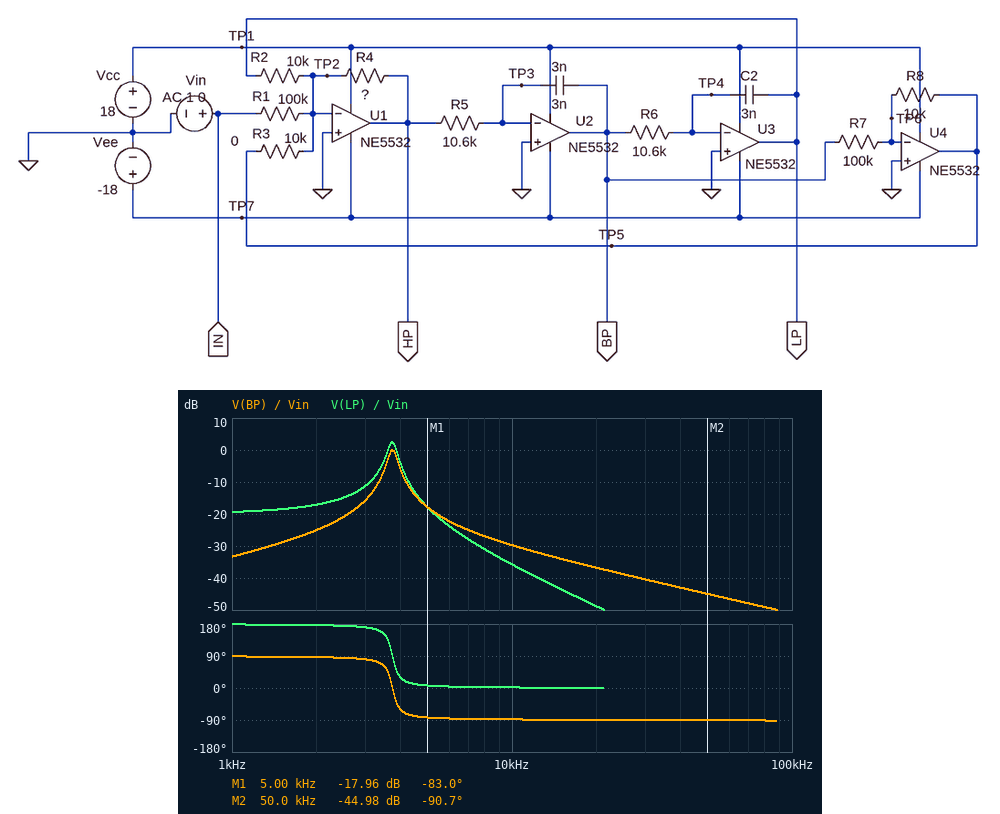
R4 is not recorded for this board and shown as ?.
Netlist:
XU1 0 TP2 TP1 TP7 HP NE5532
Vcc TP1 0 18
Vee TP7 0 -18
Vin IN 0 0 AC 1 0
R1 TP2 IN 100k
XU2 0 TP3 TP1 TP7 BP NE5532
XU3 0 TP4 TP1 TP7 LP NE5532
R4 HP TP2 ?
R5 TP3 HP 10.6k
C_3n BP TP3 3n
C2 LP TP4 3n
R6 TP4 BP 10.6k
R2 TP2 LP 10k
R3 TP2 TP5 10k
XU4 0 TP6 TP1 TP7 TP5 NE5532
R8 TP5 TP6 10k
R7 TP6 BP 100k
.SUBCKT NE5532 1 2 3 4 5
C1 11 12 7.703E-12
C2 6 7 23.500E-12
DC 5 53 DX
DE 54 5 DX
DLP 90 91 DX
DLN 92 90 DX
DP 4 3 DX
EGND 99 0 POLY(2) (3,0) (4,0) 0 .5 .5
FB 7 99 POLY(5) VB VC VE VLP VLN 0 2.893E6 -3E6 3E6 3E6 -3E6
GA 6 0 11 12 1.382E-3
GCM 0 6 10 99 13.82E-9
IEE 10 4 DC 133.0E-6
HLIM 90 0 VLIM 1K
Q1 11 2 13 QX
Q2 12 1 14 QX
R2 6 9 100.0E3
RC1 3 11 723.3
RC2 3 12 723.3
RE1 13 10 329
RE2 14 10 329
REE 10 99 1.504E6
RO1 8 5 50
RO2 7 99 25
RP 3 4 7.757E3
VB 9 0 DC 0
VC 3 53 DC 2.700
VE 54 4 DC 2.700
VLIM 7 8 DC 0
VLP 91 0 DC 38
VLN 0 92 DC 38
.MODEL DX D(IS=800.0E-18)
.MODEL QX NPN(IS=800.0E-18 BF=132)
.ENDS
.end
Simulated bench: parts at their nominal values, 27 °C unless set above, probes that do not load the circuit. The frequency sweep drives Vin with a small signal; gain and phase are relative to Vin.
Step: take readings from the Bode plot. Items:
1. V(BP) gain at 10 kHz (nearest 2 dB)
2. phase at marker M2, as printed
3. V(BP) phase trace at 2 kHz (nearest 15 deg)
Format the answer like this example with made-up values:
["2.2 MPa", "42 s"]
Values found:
["-30 dB", "-90.7 deg", "90 deg"]
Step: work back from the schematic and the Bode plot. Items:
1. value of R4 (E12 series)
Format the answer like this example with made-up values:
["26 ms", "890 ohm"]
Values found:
["5.6 kΩ"]
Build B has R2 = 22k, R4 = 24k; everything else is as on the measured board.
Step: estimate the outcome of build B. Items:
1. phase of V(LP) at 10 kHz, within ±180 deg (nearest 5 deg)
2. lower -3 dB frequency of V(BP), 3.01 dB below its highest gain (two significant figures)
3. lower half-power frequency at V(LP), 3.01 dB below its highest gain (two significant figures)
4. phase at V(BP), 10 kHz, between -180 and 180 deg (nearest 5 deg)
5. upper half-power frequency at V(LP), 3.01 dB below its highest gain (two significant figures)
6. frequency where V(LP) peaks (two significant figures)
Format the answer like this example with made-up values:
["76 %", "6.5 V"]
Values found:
["10 deg", "4.7 kHz", "4.5 kHz", "-80 deg", "5.7 kHz", "5.2 kHz"]
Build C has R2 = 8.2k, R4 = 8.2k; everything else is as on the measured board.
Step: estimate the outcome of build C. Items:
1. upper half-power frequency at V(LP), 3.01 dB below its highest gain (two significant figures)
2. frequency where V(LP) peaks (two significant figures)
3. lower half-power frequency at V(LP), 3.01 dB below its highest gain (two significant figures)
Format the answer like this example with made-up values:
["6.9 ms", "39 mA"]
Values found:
["5.2 kHz", "5.0 kHz", "4.8 kHz"]
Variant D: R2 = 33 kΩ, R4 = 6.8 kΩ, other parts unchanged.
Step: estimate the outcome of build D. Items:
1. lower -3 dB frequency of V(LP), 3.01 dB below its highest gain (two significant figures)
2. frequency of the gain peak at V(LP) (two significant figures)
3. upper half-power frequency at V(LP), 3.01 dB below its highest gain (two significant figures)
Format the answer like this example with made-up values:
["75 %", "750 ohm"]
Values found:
["2.1 kHz", "2.3 kHz", "2.4 kHz"]
